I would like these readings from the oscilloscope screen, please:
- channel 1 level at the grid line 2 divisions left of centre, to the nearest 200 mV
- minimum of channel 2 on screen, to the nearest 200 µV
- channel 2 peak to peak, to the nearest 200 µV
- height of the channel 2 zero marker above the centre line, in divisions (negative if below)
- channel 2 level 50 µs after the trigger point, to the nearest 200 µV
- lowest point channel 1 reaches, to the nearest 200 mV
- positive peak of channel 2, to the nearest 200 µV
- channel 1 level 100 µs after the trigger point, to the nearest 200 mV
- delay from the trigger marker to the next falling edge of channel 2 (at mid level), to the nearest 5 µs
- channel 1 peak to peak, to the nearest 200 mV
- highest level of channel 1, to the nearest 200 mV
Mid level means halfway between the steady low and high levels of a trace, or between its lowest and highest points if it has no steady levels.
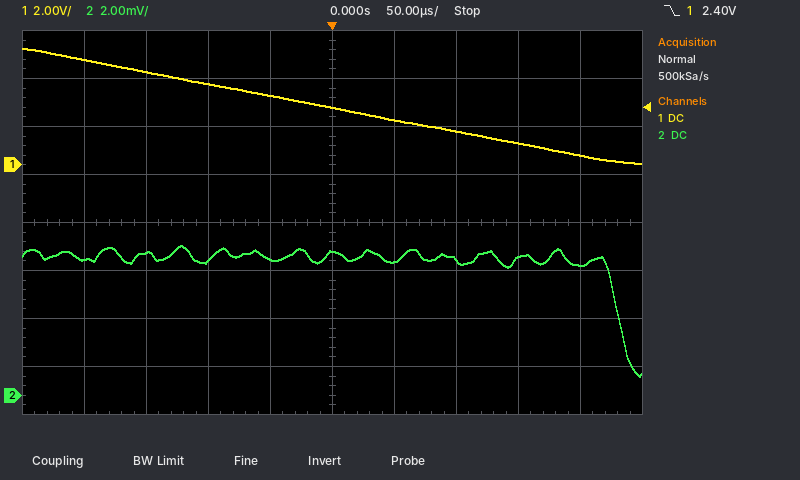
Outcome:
3.4 V
800 µV
5.4 mV
-3.6 div
5.6 mV
0.0 V
6.2 mV
1.4 V
230 µs
4.8 V
4.8 V
